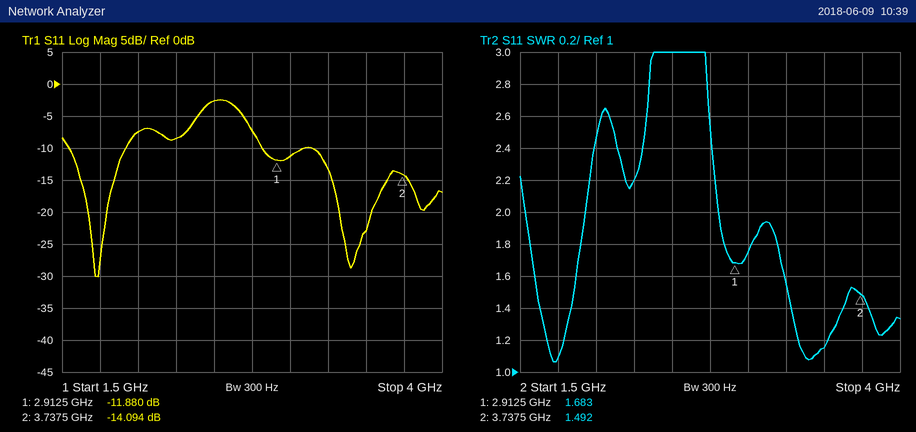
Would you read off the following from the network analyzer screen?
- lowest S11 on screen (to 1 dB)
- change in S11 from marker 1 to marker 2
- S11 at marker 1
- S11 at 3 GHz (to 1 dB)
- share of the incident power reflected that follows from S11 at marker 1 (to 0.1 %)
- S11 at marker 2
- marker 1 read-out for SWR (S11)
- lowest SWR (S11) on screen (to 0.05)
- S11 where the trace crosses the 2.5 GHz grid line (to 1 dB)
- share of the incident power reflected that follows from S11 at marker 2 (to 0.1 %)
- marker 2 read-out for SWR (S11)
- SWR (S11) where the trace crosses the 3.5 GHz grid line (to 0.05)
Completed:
-30 dB
-2.214 dB
-11.880 dB
-11 dB
6.5 %
-14.094 dB
1.683
1.05
-3 dB
3.9 %
1.492
1.15
